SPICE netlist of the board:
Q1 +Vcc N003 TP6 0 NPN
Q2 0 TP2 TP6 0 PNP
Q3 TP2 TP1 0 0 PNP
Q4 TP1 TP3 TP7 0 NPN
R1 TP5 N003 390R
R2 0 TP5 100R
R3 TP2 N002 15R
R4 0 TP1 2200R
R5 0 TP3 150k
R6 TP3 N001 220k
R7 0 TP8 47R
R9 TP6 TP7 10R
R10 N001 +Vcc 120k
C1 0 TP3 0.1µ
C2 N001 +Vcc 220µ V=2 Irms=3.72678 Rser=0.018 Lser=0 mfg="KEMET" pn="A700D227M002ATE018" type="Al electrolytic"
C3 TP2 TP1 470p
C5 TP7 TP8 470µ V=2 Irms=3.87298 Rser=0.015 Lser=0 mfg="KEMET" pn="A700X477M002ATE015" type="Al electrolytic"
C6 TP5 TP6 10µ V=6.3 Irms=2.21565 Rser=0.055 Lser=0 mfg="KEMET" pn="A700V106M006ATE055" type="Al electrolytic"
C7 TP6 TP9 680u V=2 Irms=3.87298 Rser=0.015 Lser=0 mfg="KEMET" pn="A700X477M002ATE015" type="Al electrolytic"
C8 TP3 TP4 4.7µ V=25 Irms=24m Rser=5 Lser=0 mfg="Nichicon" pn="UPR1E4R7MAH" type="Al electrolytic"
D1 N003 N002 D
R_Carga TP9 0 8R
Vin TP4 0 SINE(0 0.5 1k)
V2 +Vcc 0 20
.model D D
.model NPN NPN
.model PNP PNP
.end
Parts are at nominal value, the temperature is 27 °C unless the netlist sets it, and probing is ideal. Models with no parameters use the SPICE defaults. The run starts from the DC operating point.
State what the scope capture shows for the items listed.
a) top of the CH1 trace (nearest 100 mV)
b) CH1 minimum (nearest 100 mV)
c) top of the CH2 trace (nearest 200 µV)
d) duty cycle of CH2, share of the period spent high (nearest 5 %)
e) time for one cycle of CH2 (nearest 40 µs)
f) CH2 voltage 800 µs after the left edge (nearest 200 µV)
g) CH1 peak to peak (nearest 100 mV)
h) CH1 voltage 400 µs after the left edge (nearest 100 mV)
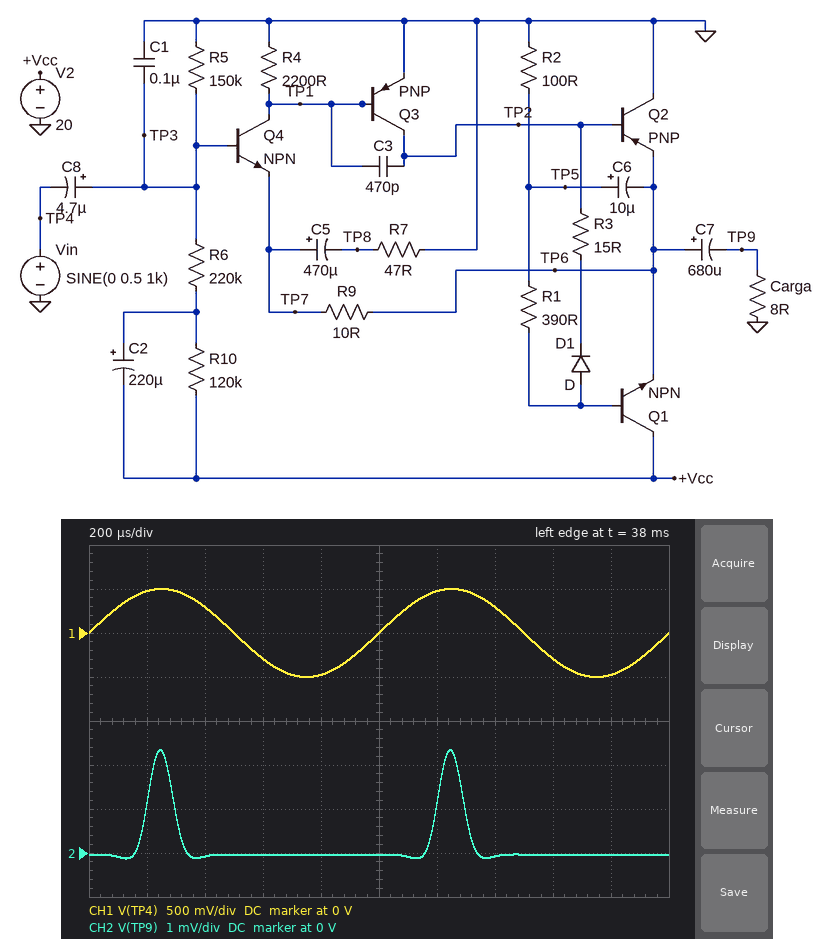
500 mV
-500 mV
2.4 mV
10 %
1.00 ms
0 V
1.0 V
300 mV
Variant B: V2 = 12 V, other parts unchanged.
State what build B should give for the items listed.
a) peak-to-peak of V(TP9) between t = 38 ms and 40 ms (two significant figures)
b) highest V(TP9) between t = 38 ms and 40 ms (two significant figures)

1.5 mV
1.4 mV
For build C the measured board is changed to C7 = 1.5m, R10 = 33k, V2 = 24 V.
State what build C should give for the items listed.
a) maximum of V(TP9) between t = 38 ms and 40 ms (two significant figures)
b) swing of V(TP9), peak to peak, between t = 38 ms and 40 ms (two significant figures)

3.7 mV
3.8 mV
